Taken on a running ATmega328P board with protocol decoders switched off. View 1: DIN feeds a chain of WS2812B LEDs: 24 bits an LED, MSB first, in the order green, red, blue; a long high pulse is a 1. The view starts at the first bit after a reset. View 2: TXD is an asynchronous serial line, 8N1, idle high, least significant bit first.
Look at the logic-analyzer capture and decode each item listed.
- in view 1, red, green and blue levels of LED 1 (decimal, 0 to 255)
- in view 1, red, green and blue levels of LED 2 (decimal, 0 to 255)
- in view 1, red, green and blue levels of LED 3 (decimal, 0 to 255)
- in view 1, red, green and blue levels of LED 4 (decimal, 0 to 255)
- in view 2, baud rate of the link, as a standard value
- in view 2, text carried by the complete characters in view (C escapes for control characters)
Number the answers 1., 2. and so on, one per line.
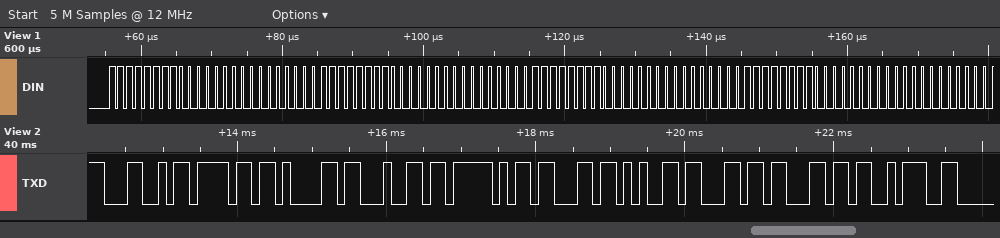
1. 0, 255, 0
2. 0, 255, 0
3. 0, 255, 0
4. 0, 255, 0
5. 9600 baud
6. "Load_cell:"
